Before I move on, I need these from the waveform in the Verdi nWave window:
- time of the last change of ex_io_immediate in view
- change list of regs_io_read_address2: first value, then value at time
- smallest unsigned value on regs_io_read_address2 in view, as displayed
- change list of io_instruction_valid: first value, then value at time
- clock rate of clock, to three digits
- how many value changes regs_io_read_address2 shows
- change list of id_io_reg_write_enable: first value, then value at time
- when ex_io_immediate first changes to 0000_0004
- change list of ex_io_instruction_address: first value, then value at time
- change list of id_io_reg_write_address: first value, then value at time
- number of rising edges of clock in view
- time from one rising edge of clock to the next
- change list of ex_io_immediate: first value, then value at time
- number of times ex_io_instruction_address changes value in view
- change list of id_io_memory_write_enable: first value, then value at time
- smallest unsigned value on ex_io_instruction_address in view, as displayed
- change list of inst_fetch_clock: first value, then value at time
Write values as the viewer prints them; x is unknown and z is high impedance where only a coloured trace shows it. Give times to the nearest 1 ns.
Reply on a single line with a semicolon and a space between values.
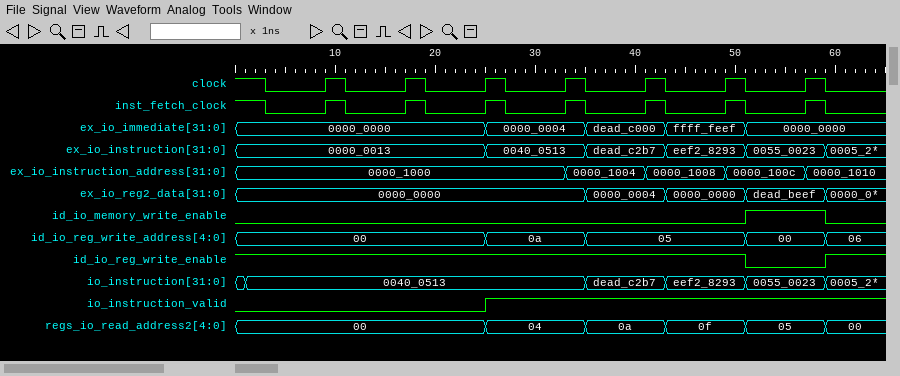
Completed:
51 ns; 00, 04 at 25 ns, 0a at 35 ns, 0f at 43 ns, 05 at 51 ns, 00 at 59 ns; 00; 0, 1 at 25 ns; 125 MHz; 5; 1, 0 at 51 ns, 1 at 59 ns; 25 ns; 0000_1000, 0000_1004 at 33 ns, 0000_1008 at 41 ns, 0000_100c at 49 ns, 0000_1010 at 57 ns; 00, 0a at 25 ns, 05 at 35 ns, 00 at 51 ns, 06 at 59 ns; 7; 8 ns; 0000_0000, 0000_0004 at 25 ns, dead_c000 at 35 ns, ffff_feef at 43 ns, 0000_0000 at 51 ns; 4; 0, 1 at 51 ns, 0 at 59 ns; 0000_1000; 1, 0 at 3 ns, 1 at 9 ns, 0 at 11 ns, 1 at 17 ns, 0 at 19 ns, 1 at 25 ns, 0 at 27 ns, 1 at 33 ns, 0 at 35 ns, 1 at 41 ns, 0 at 43 ns, 1 at 49 ns, 0 at 51 ns, 1 at 57 ns, 0 at 59 ns
